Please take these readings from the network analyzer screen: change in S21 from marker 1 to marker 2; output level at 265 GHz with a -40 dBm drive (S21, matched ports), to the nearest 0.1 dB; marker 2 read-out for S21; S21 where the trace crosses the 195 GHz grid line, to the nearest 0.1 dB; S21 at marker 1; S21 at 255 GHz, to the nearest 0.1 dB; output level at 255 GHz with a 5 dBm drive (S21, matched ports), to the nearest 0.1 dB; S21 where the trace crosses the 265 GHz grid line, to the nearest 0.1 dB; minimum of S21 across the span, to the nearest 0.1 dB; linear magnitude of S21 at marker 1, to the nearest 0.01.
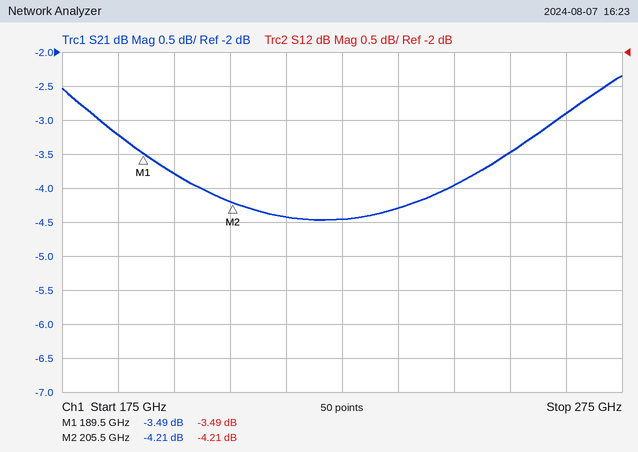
-0.72 dB
-42.9 dBm
-4.21 dB
-3.8 dB
-3.49 dB
-3.5 dB
1.5 dBm
-2.9 dB
-4.5 dB
0.67
